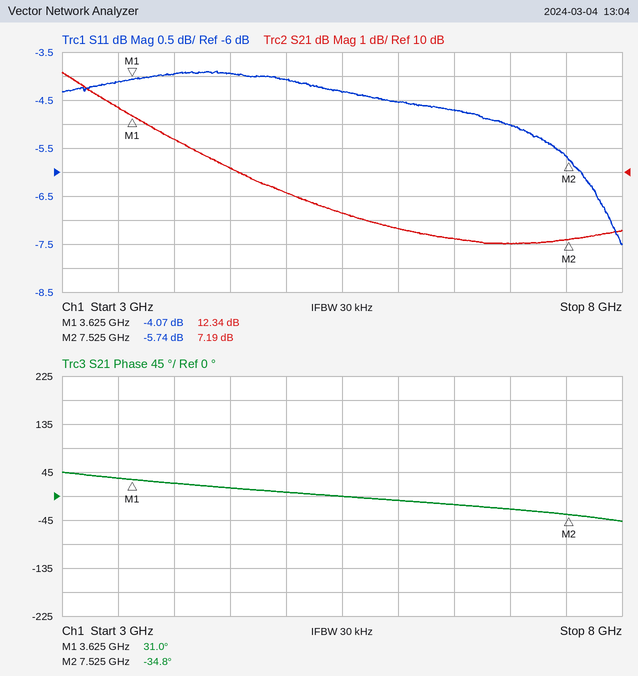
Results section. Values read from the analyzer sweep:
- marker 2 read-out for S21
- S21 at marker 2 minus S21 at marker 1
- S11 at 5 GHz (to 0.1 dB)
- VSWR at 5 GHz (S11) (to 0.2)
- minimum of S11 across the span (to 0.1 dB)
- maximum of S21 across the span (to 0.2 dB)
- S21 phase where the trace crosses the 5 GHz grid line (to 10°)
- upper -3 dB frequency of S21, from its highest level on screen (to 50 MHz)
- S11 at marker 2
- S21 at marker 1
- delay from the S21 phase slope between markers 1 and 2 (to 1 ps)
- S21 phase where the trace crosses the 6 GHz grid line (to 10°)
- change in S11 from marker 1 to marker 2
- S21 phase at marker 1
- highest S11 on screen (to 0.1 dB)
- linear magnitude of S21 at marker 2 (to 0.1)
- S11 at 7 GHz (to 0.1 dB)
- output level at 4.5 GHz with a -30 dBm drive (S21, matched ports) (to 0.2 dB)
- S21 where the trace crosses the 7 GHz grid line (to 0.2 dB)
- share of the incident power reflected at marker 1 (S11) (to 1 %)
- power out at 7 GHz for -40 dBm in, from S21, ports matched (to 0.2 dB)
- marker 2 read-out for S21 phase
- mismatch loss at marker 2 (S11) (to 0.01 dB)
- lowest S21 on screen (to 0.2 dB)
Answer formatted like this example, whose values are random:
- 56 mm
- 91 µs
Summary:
- 7.19 dB
- -5.15 dB
- -4.1 dB
- 4.4
- -7.5 dB
- 14.2 dB
- 10°
- 4.10 GHz
- -5.74 dB
- 12.34 dB
- 47 ps
- -10°
- -1.67 dB
- 31.0°
- -3.9 dB
- 2.3
- -5.0 dB
- -19.8 dBm
- 7.0 dB
- 39 %
- -33.0 dBm
- -34.8°
- 1.35 dB
- 7.0 dB
